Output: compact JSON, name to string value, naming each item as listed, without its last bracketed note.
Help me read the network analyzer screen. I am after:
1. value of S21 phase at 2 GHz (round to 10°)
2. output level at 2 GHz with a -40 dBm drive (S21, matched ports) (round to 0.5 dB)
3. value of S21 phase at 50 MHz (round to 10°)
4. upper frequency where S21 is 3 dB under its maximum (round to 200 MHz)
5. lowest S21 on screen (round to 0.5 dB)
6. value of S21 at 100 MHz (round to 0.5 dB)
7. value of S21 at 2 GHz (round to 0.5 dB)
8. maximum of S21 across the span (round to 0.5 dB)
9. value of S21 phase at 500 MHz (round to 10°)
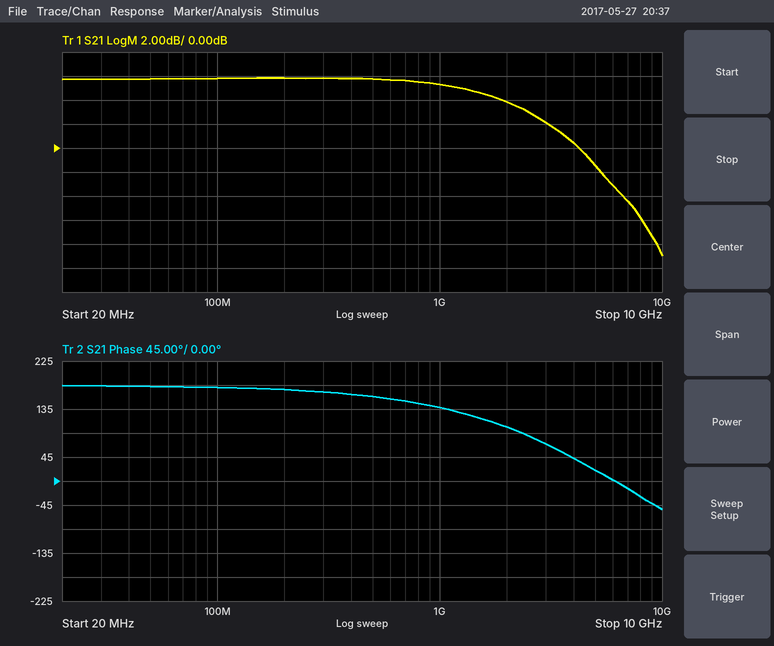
{"value of S21 phase at 2 GHz": "100°", "output level at 2 GHz with a -40 dBm drive (S21, matched ports)": "-36.0 dBm", "value of S21 phase at 50 MHz": "180°", "upper frequency where S21 is 3 dB under its maximum": "2.6 GHz", "lowest S21 on screen": "-9.0 dB", "value of S21 at 100 MHz": "6.0 dB", "value of S21 at 2 GHz": "4.0 dB", "maximum of S21 across the span": "6.0 dB", "value of S21 phase at 500 MHz": "160°"}
